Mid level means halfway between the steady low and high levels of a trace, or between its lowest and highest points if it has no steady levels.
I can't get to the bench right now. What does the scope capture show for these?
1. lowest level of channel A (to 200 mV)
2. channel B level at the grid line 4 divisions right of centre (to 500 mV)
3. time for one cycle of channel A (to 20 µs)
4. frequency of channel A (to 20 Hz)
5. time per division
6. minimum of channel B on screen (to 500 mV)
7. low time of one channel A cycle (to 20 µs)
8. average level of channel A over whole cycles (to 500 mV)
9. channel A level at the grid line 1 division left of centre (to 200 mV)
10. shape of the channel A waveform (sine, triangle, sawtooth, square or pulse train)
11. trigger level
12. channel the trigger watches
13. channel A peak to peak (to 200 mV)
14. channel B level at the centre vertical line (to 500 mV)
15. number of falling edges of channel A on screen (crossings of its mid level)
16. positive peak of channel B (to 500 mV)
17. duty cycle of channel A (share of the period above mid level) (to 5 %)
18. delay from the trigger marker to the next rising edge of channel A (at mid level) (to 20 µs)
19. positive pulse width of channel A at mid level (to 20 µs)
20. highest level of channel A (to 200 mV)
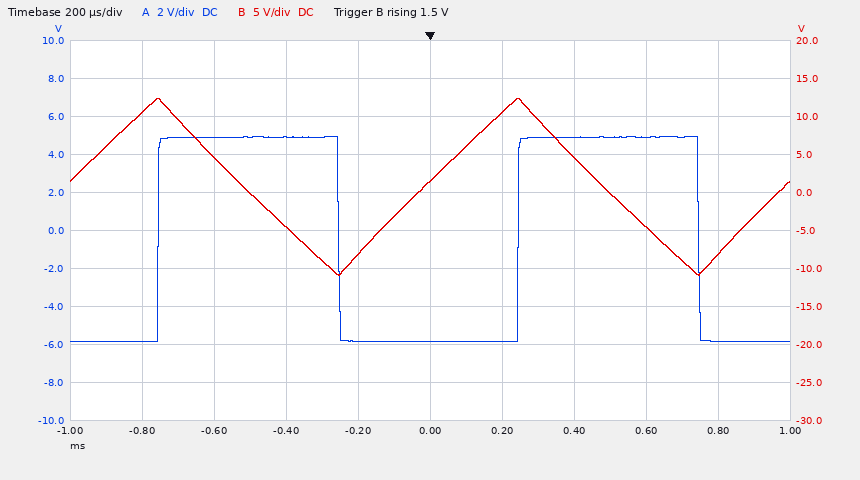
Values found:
-5.8 V
-8.0 V
1.00 ms
1.00 kHz
200 µs
-11.0 V
500 µs
-500 mV
-5.8 V
square
1.5 V
channel B
10.8 V
1.5 V
2
12.5 V
50 %
240 µs
500 µs
5.0 V
